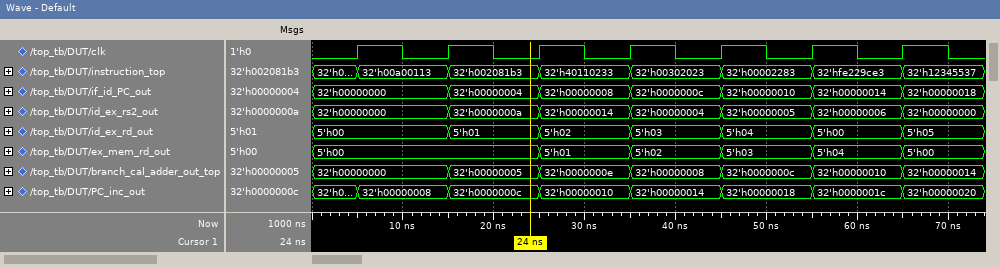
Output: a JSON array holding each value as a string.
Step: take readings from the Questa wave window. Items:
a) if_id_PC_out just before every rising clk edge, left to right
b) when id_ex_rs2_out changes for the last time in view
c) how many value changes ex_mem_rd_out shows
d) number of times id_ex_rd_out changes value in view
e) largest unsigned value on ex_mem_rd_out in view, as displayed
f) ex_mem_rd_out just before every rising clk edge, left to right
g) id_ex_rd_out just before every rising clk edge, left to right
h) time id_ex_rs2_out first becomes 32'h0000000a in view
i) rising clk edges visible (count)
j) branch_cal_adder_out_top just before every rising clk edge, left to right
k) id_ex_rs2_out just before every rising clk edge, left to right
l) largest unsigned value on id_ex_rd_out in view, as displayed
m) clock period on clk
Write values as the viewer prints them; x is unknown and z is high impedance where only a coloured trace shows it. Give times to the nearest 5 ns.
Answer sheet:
["32'h00000000, 32'h00000000, 32'h00000004, 32'h00000008, 32'h0000000c, 32'h00000010, 32'h00000014", "65 ns", "5", "6", "5'h04", "5'h00, 5'h00, 5'h00, 5'h01, 5'h02, 5'h03, 5'h04", "5'h00, 5'h00, 5'h01, 5'h02, 5'h03, 5'h04, 5'h00", "15 ns", "7", "32'h00000000, 32'h00000000, 32'h00000005, 32'h0000000e, 32'h00000008, 32'h0000000c, 32'h00000010", "32'h00000000, 32'h00000000, 32'h0000000a, 32'h00000014, 32'h00000004, 32'h00000005, 32'h00000006", "5'h05", "10 ns"]
